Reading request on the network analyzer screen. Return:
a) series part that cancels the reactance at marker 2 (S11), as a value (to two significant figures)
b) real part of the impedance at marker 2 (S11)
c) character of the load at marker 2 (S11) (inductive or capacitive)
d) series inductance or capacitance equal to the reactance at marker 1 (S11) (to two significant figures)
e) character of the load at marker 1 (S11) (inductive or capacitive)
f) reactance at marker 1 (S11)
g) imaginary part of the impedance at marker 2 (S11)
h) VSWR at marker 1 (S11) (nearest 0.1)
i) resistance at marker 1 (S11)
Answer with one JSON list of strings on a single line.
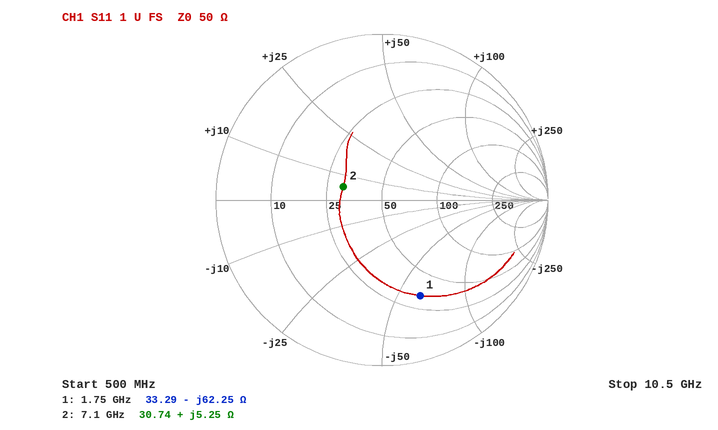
["4.3 pF", "30.74 Ω", "inductive", "1.5 pF", "capacitive", "-62.25 Ω", "+5.25 Ω", "4.3", "33.29 Ω"]
